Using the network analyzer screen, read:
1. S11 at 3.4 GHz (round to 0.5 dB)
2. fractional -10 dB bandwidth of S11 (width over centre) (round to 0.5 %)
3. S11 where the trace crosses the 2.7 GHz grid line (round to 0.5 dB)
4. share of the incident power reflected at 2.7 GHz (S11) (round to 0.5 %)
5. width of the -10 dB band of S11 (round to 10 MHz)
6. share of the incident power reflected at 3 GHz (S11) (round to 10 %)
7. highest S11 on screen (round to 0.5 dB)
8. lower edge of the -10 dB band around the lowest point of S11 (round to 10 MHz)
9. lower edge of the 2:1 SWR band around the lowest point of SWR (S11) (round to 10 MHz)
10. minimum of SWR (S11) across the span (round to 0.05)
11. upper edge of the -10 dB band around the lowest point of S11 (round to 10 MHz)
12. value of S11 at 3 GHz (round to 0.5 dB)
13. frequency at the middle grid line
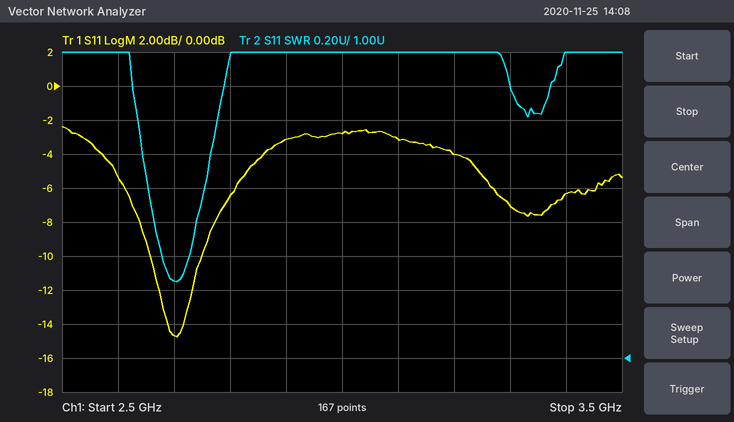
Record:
-6.5 dB
3.5 %
-14.5 dB
3.5 %
90 MHz
50 %
-2.5 dB
2.66 GHz
2.65 GHz
1.45
2.75 GHz
-3.0 dB
3 GHz
